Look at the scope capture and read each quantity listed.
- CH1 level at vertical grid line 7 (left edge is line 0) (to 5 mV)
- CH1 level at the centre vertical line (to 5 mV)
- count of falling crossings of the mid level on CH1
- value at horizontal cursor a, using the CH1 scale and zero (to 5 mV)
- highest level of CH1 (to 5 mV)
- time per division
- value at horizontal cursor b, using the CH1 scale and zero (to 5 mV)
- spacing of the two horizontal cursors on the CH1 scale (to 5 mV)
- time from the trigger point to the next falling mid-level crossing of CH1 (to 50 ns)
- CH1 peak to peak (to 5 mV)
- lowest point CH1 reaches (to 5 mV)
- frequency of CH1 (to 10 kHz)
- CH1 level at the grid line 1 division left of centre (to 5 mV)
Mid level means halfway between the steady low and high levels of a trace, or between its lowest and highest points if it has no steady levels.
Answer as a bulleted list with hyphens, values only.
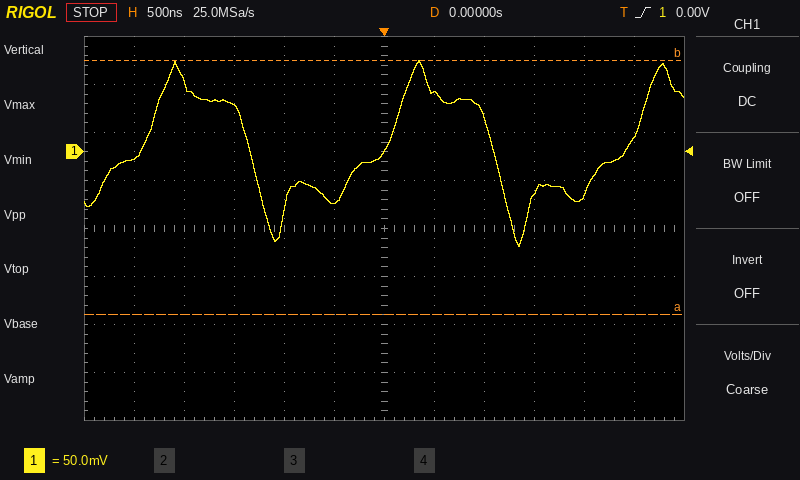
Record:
- 60 mV
- 0 mV
- 2
- -170 mV
- 95 mV
- 500 ns
- 95 mV
- 265 mV
- 1.10 µs
- 195 mV
- -100 mV
- 410 kHz
- -55 mV
